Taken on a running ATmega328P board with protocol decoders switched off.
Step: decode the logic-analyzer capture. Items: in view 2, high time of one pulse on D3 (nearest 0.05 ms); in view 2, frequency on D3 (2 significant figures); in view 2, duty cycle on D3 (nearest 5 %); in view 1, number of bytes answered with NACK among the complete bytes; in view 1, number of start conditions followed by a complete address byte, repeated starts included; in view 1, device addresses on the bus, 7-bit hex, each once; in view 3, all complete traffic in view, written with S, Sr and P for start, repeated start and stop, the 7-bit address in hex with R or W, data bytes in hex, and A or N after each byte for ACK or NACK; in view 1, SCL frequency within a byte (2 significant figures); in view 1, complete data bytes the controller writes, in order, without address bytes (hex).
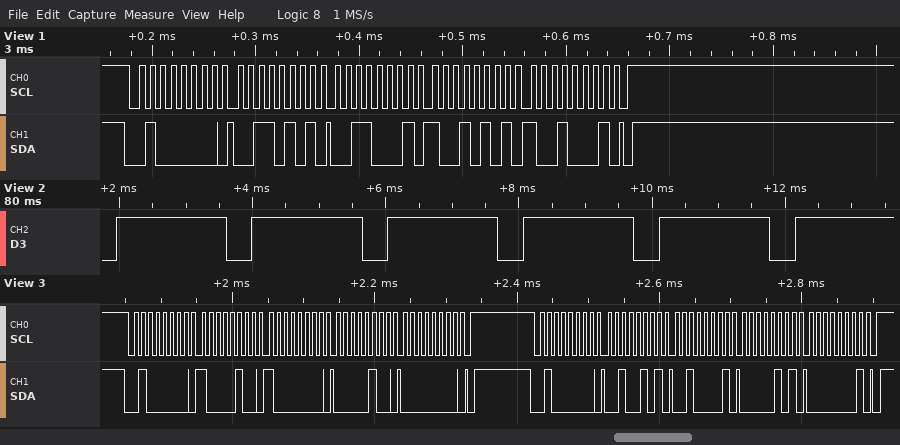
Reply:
1.65 ms
490 Hz
80 %
0
1
0x20
S 20W A 84 A 80 A 04 A 00 A P S 20W A 25 A 21 A 05 A 01 A P
100 kHz
35 31 95 91
